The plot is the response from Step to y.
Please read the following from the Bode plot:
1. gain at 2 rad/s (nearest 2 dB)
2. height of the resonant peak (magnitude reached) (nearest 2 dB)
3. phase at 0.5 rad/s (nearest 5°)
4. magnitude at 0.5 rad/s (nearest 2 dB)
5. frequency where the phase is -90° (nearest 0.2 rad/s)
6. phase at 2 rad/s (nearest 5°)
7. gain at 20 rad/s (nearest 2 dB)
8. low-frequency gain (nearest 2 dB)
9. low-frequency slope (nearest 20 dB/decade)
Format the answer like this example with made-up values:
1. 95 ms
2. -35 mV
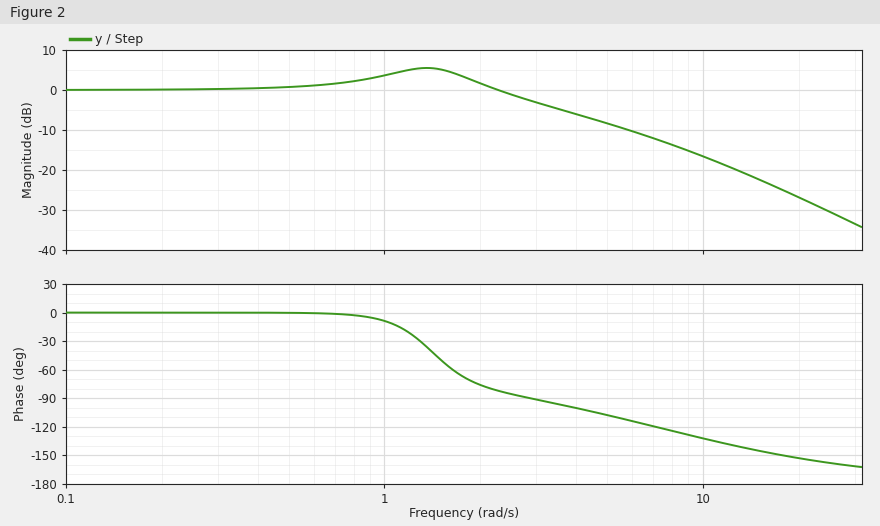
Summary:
1. 2 dB
2. 6 dB
3. 0°
4. 0 dB
5. 2.8 rad/s
6. -75°
7. -26 dB
8. 0 dB
9. 0 dB/decade
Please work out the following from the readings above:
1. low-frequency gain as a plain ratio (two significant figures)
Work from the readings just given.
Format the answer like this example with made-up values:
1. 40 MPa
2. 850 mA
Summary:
1. 1.0
